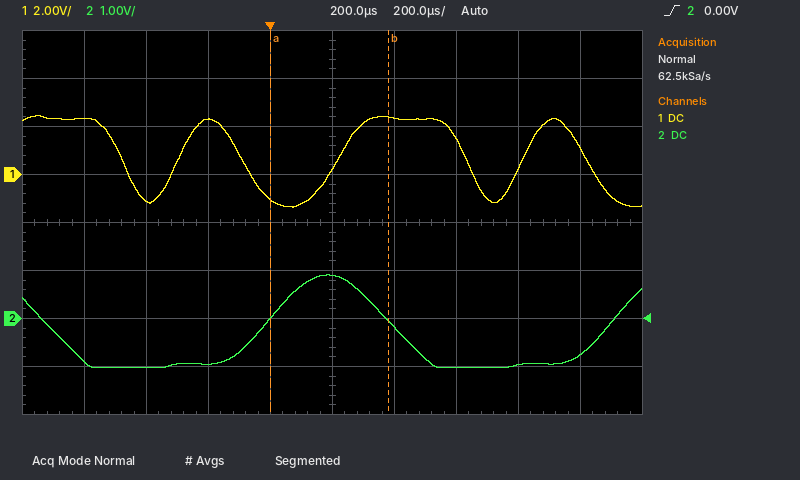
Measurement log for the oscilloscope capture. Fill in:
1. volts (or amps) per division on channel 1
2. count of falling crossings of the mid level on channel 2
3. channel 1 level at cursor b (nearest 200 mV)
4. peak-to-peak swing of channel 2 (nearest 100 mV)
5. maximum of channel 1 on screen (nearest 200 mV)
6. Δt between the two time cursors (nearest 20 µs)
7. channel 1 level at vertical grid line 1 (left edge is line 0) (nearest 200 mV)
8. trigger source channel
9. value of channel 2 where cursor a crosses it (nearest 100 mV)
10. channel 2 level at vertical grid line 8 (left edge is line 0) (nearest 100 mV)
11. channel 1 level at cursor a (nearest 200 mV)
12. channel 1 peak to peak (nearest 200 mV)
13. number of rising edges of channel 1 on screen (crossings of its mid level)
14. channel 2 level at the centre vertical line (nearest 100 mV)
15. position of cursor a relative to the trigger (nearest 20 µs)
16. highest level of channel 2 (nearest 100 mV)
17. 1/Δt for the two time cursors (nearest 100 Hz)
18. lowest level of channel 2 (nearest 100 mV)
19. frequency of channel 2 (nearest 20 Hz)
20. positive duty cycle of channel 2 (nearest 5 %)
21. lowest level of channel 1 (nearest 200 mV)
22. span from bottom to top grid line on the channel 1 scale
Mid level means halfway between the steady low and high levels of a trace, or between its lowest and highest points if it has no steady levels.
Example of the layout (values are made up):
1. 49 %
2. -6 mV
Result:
1. 2 V
2. 2
3. 2.4 V
4. 1.9 V
5. 2.4 V
6. 380 µs
7. 2.4 V
8. channel 2
9. 0.0 V
10. -1.0 V
11. -1.0 V
12. 3.8 V
13. 3
14. 900 mV
15. 0 µs
16. 900 mV
17. 2.6 kHz
18. -1.0 V
19. 900 Hz
20. 35 %
21. -1.4 V
22. 16 V
